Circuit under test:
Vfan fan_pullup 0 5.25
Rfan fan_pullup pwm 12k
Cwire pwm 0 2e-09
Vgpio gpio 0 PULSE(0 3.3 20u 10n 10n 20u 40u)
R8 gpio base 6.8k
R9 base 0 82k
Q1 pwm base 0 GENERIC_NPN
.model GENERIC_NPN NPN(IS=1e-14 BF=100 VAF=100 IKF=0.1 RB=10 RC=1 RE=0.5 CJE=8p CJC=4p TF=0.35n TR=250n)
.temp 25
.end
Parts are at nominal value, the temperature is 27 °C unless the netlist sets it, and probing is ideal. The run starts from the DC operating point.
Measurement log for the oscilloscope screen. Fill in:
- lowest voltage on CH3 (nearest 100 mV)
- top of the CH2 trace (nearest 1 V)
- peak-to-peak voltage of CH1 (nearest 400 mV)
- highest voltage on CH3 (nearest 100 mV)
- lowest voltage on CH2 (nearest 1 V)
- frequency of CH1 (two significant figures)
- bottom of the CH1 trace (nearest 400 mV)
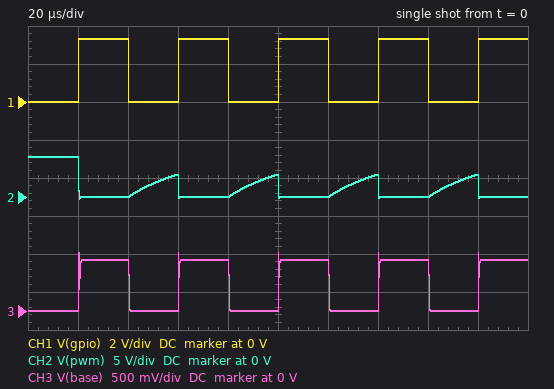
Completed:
0 V
5 V
3.2 V
800 mV
0 V
25 kHz
0 V
